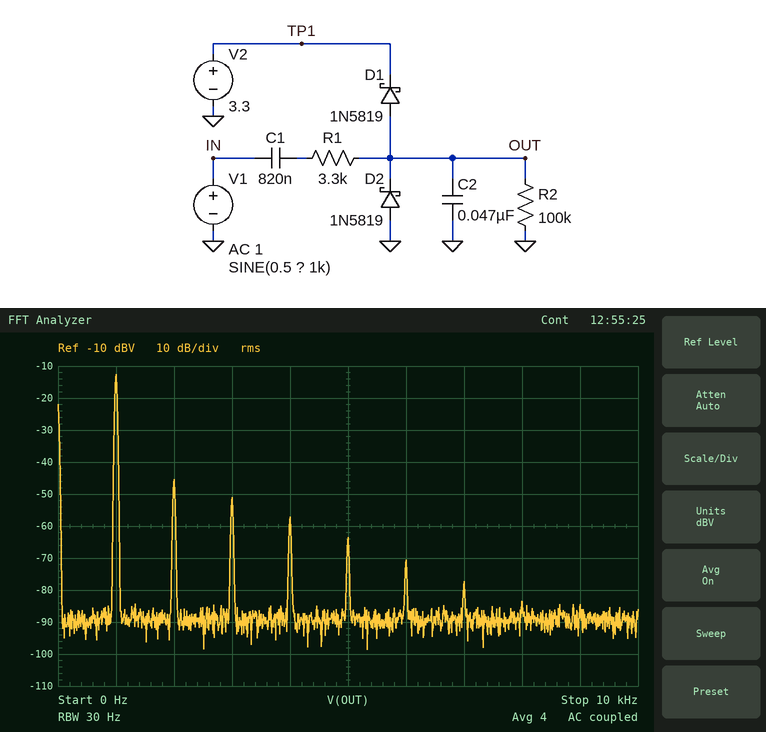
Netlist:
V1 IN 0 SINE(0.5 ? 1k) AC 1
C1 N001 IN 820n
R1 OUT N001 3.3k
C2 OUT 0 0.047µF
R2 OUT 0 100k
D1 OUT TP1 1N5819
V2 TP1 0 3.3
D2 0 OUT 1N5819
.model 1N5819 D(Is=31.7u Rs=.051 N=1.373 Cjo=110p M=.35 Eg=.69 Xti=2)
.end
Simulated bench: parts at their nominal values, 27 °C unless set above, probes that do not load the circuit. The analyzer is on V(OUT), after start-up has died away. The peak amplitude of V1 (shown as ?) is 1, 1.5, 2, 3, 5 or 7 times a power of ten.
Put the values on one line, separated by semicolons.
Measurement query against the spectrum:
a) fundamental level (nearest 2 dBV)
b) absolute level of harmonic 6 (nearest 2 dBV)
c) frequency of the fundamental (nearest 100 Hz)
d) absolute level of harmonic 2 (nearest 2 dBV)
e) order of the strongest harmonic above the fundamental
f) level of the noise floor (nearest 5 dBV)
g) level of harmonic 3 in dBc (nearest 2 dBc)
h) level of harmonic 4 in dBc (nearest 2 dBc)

-12 dBV; -70 dBV; 1.0 kHz; -46 dBV; 2; -90 dBV; -38 dBc; -44 dBc
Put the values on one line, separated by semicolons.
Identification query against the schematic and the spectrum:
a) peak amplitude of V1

500 mV
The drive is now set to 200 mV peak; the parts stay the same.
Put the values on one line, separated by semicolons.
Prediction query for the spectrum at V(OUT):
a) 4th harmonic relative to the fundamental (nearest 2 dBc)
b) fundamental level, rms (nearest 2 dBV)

-54 dBc; -20 dBV
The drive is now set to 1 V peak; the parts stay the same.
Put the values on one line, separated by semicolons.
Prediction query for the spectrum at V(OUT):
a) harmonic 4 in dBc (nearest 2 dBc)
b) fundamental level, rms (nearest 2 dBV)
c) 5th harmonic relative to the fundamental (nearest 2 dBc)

-42 dBc; -6 dBV; -46 dBc
